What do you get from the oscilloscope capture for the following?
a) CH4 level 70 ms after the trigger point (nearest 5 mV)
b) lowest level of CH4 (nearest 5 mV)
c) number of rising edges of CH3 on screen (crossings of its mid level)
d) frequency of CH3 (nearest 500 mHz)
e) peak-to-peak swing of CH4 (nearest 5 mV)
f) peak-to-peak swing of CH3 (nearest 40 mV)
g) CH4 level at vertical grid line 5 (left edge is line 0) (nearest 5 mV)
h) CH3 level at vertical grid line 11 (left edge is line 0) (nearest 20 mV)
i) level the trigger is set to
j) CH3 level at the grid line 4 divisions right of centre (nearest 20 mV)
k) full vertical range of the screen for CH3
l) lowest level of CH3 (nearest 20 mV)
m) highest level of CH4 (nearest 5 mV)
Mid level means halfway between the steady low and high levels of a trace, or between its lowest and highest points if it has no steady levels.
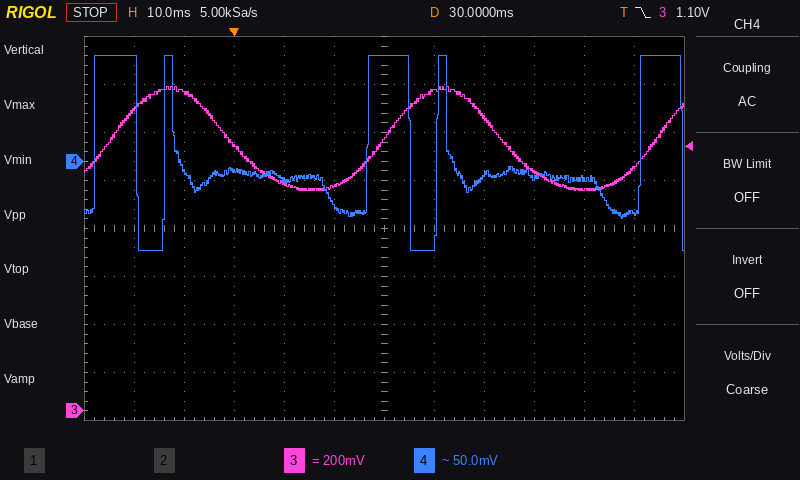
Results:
-20 mV
-95 mV
3
18.5 Hz
205 mV
440 mV
-45 mV
1.02 V
1.10 V
920 mV
1.6 V
920 mV
110 mV
